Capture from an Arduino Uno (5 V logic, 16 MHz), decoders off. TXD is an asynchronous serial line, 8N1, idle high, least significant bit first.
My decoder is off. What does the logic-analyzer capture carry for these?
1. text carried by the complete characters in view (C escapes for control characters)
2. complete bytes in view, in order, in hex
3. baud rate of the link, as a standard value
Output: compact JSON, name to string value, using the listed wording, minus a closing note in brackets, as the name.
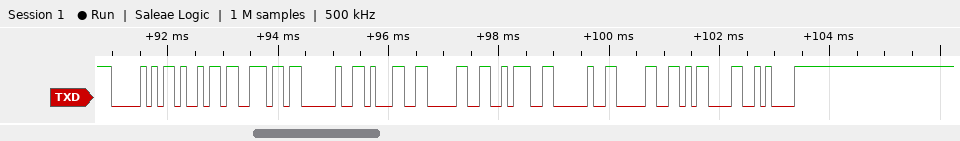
{"text carried by the complete characters in view": "\"Pin 10: 0\\r\\n\"", "complete bytes in view, in order, in hex": "0x50 0x69 0x6E 0x20 0x31 0x30 0x3A 0x20 0x30 0x0D 0x0A", "baud rate of the link, as a standard value": "9600 baud"}
